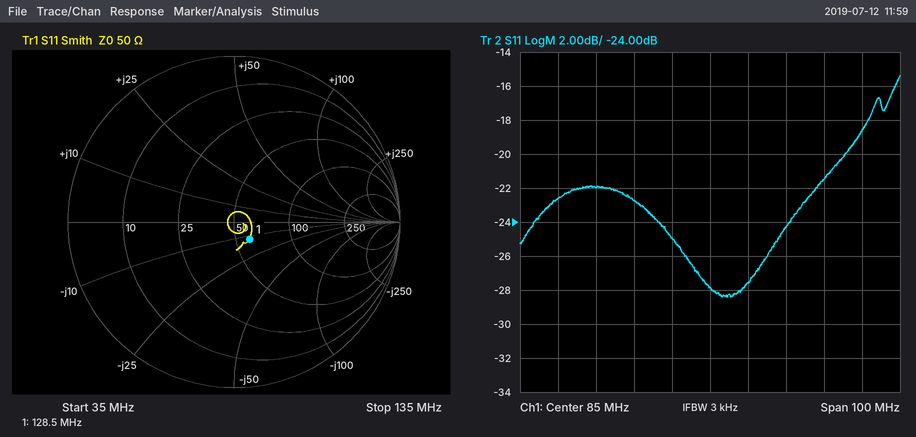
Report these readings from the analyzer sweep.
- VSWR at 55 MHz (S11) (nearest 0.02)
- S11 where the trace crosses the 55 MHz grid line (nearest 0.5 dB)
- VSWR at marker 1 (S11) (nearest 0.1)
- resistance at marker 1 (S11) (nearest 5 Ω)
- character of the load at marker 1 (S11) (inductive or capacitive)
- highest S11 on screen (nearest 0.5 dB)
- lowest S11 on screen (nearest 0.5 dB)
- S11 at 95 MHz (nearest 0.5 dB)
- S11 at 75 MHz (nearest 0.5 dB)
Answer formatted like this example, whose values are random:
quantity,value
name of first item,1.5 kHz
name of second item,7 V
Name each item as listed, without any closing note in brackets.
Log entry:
quantity,value
VSWR at 55 MHz (S11),1.18
S11 where the trace crosses the 55 MHz grid line,-22.0 dB
VSWR at marker 1 (S11),1.3
resistance at marker 1 (S11),60 Ω
character of the load at marker 1 (S11),capacitive
highest S11 on screen,-15.5 dB
lowest S11 on screen,-28.5 dB
S11 at 95 MHz,-27.5 dB
S11 at 75 MHz,-25.0 dB
